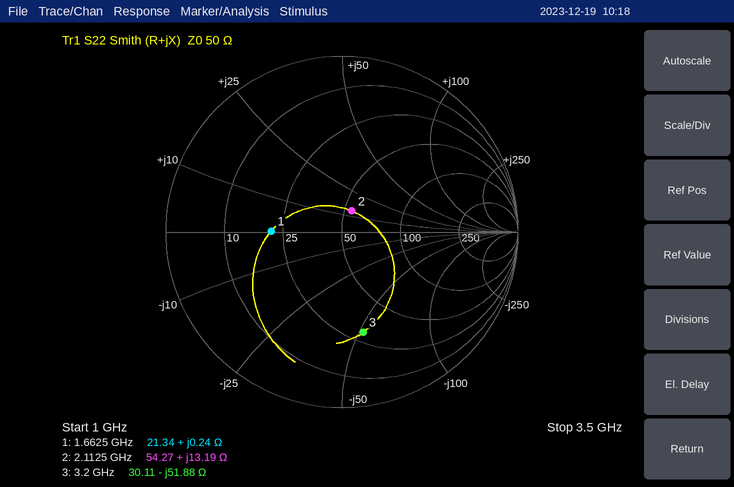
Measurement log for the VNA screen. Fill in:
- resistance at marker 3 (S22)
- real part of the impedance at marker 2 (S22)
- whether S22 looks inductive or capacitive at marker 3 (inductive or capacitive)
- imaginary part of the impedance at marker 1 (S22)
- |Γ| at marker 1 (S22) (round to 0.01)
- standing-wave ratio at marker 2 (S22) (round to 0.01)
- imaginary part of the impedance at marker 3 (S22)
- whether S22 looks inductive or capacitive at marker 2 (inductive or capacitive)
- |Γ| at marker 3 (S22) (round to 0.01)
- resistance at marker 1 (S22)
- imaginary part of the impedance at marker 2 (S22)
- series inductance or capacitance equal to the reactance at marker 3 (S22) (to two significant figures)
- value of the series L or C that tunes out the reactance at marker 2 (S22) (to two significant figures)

30.11 Ω
54.27 Ω
capacitive
+0.24 Ω
0.40
1.30
-51.88 Ω
inductive
0.58
21.34 Ω
+13.19 Ω
960 fF
5.7 pF
